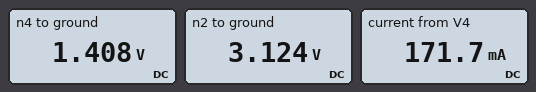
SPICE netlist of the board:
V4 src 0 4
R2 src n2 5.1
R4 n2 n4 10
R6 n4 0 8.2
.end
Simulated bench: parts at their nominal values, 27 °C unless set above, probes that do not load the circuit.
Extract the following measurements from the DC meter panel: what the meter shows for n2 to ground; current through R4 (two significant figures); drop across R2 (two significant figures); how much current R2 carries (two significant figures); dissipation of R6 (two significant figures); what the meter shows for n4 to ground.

3.124 V
170 mA
880 mV
170 mA
240 mW
1.408 V
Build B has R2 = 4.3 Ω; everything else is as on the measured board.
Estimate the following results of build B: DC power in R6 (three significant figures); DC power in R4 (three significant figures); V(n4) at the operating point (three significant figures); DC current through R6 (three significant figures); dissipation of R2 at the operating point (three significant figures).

259 mW
316 mW
1.46 V
178 mA
136 mW
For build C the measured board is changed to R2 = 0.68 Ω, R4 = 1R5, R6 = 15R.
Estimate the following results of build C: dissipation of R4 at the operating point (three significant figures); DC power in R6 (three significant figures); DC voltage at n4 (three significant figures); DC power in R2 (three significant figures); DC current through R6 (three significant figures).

81.3 mW
813 mW
3.49 V
36.9 mW
233 mA
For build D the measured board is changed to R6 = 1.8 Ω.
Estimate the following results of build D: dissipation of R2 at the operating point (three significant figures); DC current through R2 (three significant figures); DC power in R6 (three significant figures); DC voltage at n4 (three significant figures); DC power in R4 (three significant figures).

286 mW
237 mA
101 mW
426 mV
560 mW
